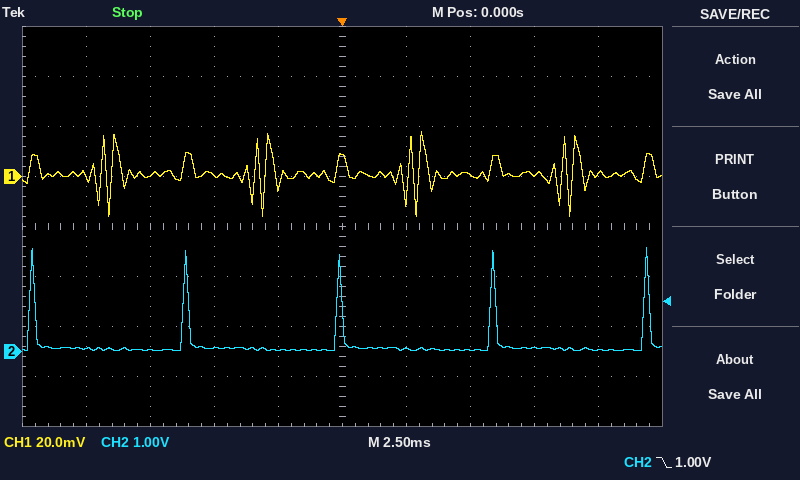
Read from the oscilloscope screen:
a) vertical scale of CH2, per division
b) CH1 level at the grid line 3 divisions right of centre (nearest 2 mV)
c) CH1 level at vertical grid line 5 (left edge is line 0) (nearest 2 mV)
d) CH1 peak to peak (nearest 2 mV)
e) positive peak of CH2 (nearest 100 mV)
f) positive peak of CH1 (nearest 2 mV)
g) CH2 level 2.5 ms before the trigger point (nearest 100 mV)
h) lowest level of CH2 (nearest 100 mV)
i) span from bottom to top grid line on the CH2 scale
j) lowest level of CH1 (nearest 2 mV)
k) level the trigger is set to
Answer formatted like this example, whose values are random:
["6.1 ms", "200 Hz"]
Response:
["1 V", "0 mV", "8 mV", "34 mV", "2.1 V", "18 mV", "0.0 V", "0.0 V", "8 V", "-16 mV", "1.00 V"]
